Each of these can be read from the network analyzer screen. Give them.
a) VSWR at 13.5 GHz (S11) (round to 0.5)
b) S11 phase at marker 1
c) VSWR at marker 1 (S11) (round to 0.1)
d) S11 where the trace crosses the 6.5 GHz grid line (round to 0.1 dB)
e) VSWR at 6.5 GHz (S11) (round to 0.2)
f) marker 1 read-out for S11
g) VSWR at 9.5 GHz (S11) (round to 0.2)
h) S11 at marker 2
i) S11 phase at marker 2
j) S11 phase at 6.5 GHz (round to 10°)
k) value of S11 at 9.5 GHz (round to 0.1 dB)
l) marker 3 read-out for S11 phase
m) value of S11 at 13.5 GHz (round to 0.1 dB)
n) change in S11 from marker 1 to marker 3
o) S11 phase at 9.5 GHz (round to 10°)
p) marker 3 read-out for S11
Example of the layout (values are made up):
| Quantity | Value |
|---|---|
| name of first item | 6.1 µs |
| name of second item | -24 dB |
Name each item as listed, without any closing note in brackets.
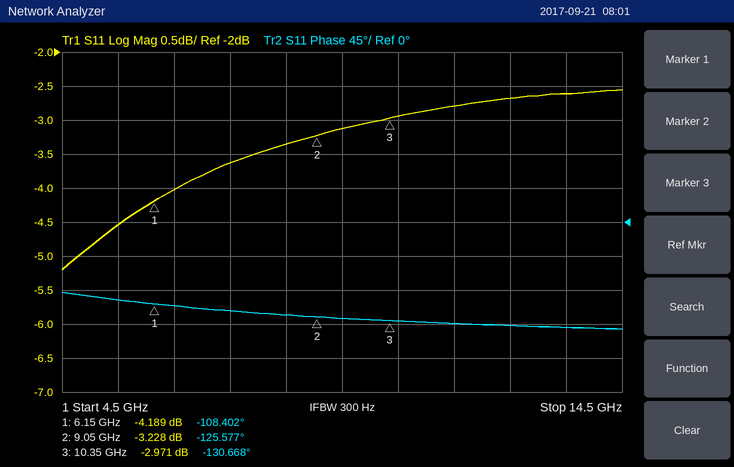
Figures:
| Quantity | Value |
|---|---|
| VSWR at 13.5 GHz (S11) | 6.5 |
| S11 phase at marker 1 | -108.402° |
| VSWR at marker 1 (S11) | 4.2 |
| S11 where the trace crosses the 6.5 GHz grid line | -4.0 dB |
| VSWR at 6.5 GHz (S11) | 4.4 |
| marker 1 read-out for S11 | -4.189 dB |
| VSWR at 9.5 GHz (S11) | 5.6 |
| S11 at marker 2 | -3.228 dB |
| S11 phase at marker 2 | -125.577° |
| S11 phase at 6.5 GHz | -110° |
| value of S11 at 9.5 GHz | -3.1 dB |
| marker 3 read-out for S11 phase | -130.668° |
| value of S11 at 13.5 GHz | -2.6 dB |
| change in S11 from marker 1 to marker 3 | 1.218 dB |
| S11 phase at 9.5 GHz | -130° |
| marker 3 read-out for S11 | -2.971 dB |
